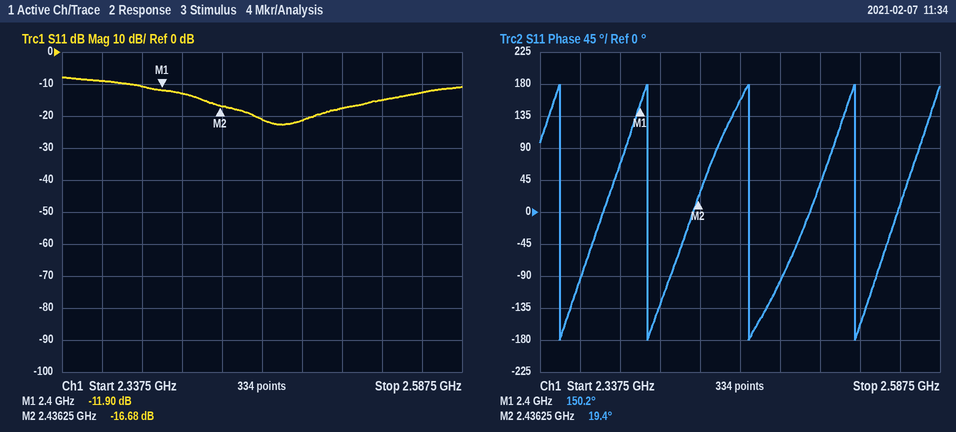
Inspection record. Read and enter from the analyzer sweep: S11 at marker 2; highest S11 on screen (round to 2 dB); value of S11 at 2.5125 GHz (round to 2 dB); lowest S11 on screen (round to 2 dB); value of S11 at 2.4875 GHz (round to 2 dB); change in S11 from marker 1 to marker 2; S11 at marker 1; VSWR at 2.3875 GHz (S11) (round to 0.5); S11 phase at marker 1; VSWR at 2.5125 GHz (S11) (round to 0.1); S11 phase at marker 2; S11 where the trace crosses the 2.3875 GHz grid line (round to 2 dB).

-16.68 dB
-8 dB
-18 dB
-22 dB
-22 dB
-4.78 dB
-11.90 dB
2.0
150.2°
1.3
19.4°
-10 dB
